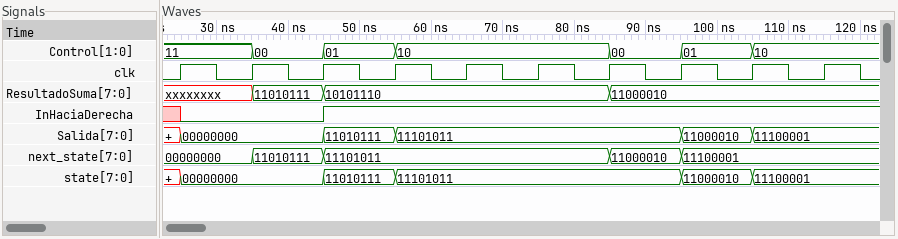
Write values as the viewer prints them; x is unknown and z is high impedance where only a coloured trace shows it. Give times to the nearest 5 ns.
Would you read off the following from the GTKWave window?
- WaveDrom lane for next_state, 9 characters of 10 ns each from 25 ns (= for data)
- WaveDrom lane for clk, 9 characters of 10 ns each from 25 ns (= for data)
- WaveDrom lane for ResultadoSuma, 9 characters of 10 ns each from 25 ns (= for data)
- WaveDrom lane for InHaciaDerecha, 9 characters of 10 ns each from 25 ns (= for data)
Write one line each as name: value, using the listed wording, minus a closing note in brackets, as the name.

WaveDrom lane for next_state, 9 characters of 10 ns each from 25 ns: {name: 'next_state', wave: '===...==.', data: '00000000 11010111 11101011 11000010 11100001'}
WaveDrom lane for clk, 9 characters of 10 ns each from 25 ns: {name: 'clk', wave: 'p........'}
WaveDrom lane for ResultadoSuma, 9 characters of 10 ns each from 25 ns: {name: 'ResultadoSuma', wave: 'x==...=..', data: '11010111 10101110 11000010'}
WaveDrom lane for InHaciaDerecha, 9 characters of 10 ns each from 25 ns: {name: 'InHaciaDerecha', wave: '0.1......'}
